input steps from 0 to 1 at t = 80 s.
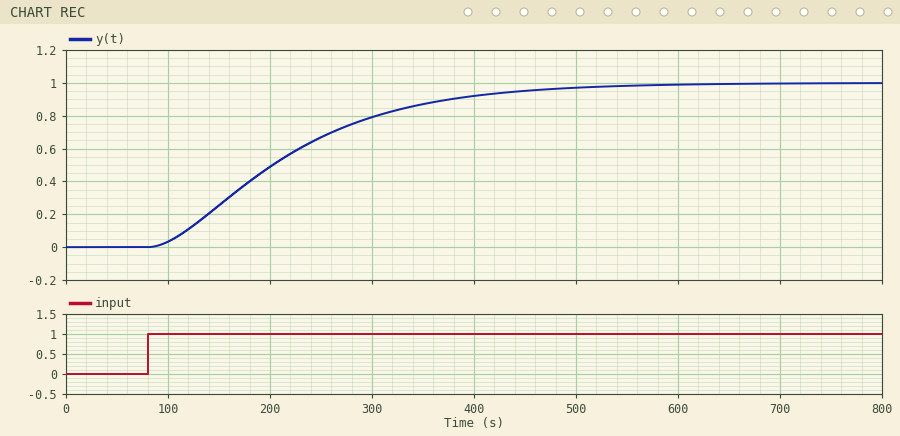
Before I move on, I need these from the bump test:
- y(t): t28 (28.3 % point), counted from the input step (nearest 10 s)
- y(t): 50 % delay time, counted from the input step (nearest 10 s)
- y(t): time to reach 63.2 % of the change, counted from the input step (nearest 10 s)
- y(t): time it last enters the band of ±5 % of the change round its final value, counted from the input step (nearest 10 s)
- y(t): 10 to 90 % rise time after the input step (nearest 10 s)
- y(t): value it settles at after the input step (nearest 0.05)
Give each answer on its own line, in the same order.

80 s
120 s
160 s
370 s
260 s
1.00
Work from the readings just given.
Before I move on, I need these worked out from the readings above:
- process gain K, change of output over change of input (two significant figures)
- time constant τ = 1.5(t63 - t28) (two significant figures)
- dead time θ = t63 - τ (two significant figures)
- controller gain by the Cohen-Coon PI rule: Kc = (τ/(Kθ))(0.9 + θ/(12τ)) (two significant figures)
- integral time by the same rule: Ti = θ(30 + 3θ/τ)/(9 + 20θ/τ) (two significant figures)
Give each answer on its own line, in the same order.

1.0
120 s
40 s
2.8
79 s
